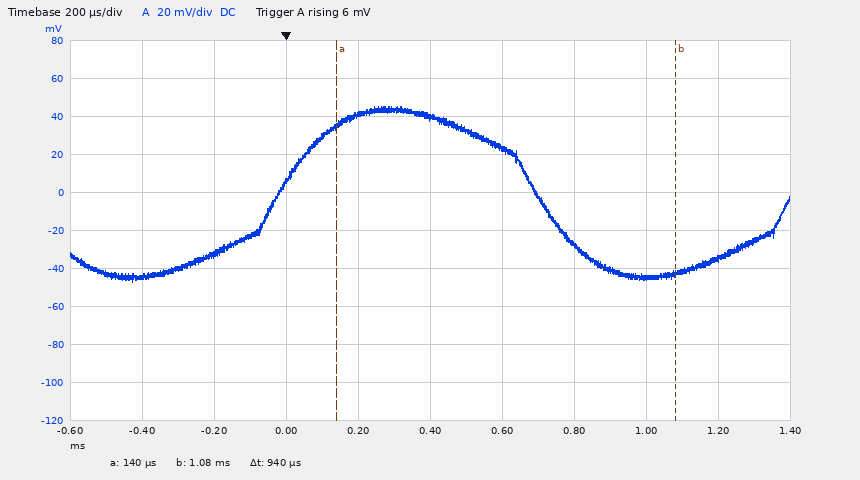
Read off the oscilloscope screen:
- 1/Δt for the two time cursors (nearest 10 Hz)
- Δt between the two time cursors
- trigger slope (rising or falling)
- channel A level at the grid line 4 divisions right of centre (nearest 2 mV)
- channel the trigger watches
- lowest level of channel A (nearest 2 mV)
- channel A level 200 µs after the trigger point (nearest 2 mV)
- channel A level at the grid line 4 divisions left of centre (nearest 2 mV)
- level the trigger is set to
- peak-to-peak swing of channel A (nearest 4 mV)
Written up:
1.06 kHz
940 µs
rising
-34 mV
channel A
-46 mV
42 mV
-44 mV
6 mV
92 mV
